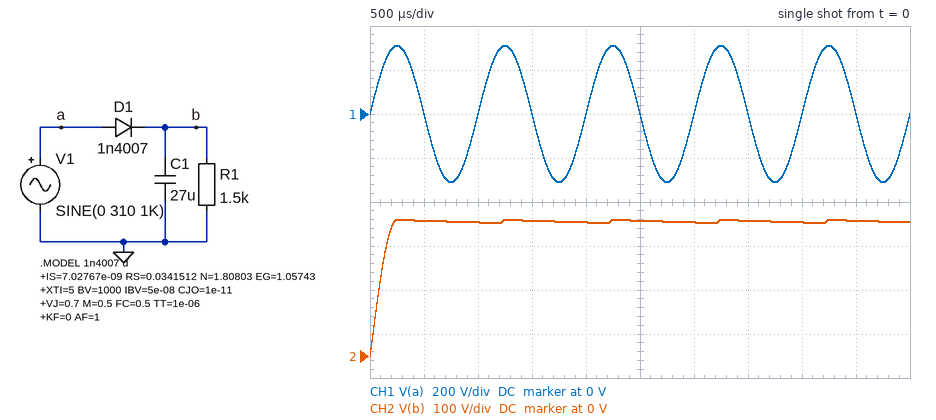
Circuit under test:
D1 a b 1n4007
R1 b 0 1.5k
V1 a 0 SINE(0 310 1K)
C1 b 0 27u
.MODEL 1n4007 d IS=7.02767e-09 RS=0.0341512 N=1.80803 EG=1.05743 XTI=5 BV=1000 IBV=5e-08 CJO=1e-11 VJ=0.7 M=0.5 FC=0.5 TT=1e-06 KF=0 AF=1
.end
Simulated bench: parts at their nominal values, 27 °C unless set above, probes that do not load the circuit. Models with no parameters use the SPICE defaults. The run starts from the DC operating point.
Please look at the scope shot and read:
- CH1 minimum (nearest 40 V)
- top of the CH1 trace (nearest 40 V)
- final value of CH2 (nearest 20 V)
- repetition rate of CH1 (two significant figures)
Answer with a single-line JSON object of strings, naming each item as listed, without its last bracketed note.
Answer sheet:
{"CH1 minimum": "-320 V", "top of the CH1 trace": "320 V", "final value of CH2": "300 V", "repetition rate of CH1": "1.0 kHz"}
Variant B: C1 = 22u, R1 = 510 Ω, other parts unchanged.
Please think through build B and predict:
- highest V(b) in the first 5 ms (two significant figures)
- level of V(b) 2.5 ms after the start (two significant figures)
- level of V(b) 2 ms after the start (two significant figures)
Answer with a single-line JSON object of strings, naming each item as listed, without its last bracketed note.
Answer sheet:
{"highest V(b) in the first 5 ms": "310 V", "level of V(b) 2.5 ms after the start": "300 V", "level of V(b) 2 ms after the start": "290 V"}
